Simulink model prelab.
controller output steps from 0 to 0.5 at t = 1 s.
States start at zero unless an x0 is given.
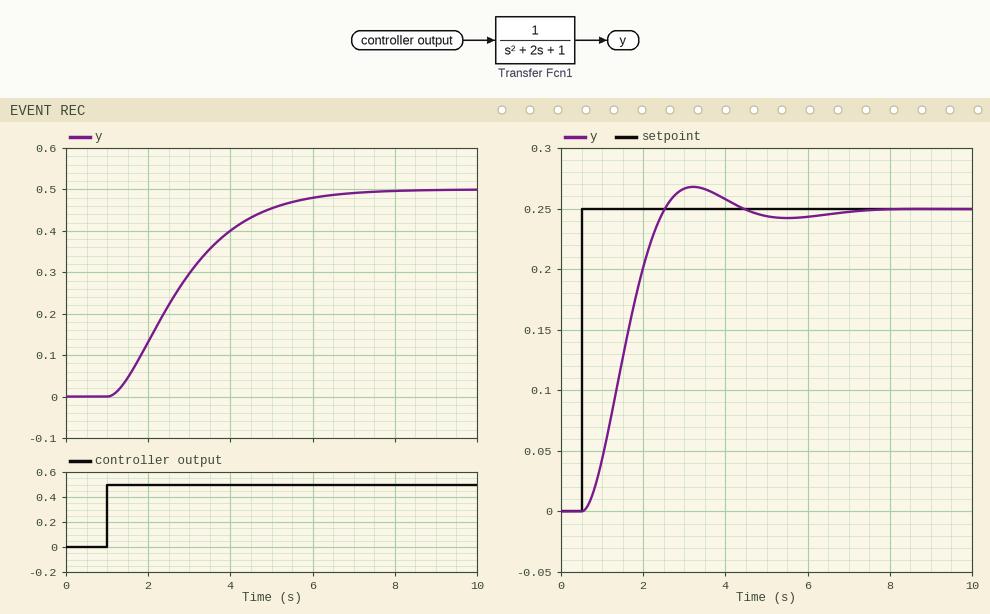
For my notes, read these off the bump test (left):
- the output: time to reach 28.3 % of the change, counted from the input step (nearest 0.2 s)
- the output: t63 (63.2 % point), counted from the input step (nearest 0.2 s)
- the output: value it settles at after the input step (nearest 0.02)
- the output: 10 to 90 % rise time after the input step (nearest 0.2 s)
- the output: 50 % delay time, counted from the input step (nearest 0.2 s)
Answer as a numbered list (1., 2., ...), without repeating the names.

1. 1.0 s
2. 2.2 s
3. 0.50
4. 3.4 s
5. 1.6 s
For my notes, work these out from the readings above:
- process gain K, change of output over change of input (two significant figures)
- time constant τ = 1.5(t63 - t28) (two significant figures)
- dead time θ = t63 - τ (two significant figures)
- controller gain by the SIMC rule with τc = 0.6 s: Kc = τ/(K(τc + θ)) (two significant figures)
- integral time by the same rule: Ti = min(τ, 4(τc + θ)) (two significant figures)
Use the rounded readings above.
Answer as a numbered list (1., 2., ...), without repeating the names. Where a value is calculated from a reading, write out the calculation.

1. (0.5 - 0) / 0.5 = 1.0
2. 1.5 × (2.2 - 1) = 1.8 s
3. 2.2 - 1.8 = 0.40 s
4. 1.8 / (1 × (0.6 + 0.4)) = 1.8
5. min(1.8, 4 × (0.6 + 0.4)) = 1.8 s
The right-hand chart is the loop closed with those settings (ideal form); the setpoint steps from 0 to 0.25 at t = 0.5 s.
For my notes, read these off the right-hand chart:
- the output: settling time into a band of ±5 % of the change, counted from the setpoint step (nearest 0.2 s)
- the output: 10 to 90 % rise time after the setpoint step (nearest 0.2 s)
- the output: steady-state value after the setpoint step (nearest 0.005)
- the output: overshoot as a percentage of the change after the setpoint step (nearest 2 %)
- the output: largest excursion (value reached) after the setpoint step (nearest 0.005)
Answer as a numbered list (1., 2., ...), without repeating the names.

1. 3.2 s
2. 1.4 s
3. 0.250
4. 8 %
5. 0.270
